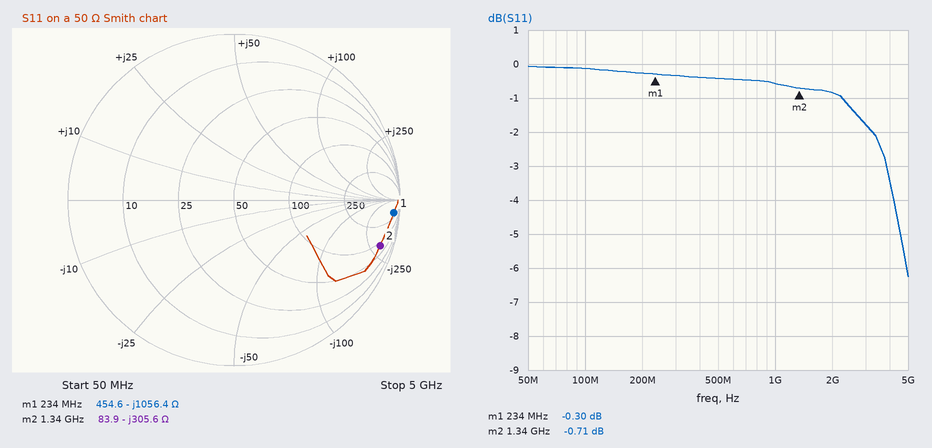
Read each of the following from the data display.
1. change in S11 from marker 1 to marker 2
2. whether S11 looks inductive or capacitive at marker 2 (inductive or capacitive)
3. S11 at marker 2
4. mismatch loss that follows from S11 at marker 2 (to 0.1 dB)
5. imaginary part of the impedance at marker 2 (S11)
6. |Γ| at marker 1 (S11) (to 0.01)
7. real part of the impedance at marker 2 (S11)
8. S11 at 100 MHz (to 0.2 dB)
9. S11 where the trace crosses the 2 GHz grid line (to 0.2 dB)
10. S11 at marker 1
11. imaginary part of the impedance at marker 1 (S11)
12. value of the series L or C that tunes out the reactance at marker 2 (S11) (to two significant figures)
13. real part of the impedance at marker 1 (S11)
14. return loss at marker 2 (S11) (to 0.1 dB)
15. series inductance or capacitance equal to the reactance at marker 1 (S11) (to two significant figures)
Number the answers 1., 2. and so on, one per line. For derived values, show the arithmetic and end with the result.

1. -0.71 − (-0.3) = -0.41 dB
2. capacitive
3. -0.71 dB
4. −10 log10(1 − 10^(-0.71/10)) ≈ 8.2 dB
5. -305.6 Ω
6. 0.97
7. 83.9 Ω
8. -0.2 dB
9. -0.8 dB
10. -0.30 dB
11. -1056.4 Ω
12. L = 305.6 Ω/(2π × 1.34 GHz) ≈ 36 nH
13. 454.6 Ω
14. 0.7 dB
15. C = 1/(2π × 234 MHz × 1056.4 Ω) ≈ 644 fF, so 640 fF to two significant figures
